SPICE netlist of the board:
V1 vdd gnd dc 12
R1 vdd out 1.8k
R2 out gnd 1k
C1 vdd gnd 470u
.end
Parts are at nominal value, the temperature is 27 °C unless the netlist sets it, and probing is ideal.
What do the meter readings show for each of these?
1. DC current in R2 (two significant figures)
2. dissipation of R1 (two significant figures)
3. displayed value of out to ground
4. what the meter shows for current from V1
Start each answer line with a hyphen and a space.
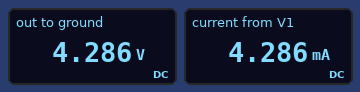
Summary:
- 4.3 mA
- 33 mW
- 4.286 V
- 4.286 mA
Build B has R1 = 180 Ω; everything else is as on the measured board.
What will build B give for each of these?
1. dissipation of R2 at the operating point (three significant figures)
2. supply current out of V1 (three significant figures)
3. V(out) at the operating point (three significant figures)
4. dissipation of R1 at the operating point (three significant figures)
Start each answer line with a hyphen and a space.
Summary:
- 103 mW
- 10.2 mA
- 10.2 V
- 18.6 mW
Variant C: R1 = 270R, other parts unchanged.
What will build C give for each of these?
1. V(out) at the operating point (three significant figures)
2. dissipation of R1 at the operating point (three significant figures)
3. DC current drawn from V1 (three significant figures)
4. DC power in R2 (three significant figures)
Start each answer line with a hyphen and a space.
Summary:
- 9.45 V
- 24.1 mW
- 9.45 mA
- 89.3 mW
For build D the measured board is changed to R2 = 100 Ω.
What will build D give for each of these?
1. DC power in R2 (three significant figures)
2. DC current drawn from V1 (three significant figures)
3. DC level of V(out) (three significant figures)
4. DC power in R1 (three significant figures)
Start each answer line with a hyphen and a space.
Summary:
- 3.99 mW
- 6.32 mA
- 632 mV
- 71.8 mW
